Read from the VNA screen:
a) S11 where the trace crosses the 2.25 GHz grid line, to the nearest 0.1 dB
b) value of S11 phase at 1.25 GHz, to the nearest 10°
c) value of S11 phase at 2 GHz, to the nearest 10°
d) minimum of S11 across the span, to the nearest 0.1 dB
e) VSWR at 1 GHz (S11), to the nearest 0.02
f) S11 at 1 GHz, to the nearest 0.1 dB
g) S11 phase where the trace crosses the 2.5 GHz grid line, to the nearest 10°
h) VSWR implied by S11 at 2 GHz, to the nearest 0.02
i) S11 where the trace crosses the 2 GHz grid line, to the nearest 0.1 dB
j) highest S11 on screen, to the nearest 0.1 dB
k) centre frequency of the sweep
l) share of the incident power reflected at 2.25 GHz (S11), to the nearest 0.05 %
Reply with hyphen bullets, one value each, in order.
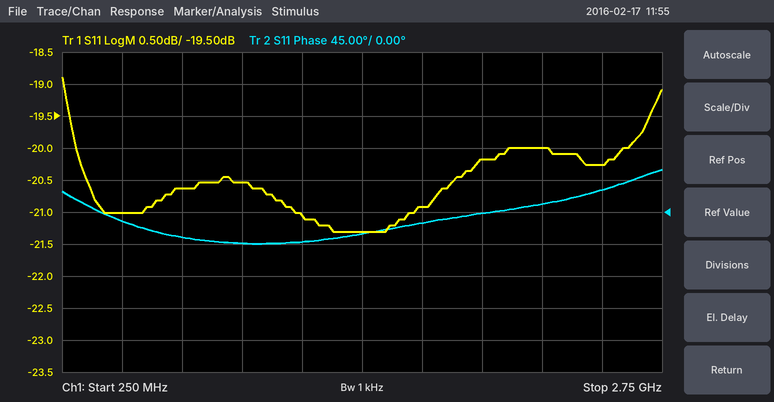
- -20.0 dB
- -40°
- 0°
- -21.3 dB
- 1.20
- -20.5 dB
- 30°
- 1.22
- -20.2 dB
- -18.9 dB
- 1.5 GHz
- 1.00 %
